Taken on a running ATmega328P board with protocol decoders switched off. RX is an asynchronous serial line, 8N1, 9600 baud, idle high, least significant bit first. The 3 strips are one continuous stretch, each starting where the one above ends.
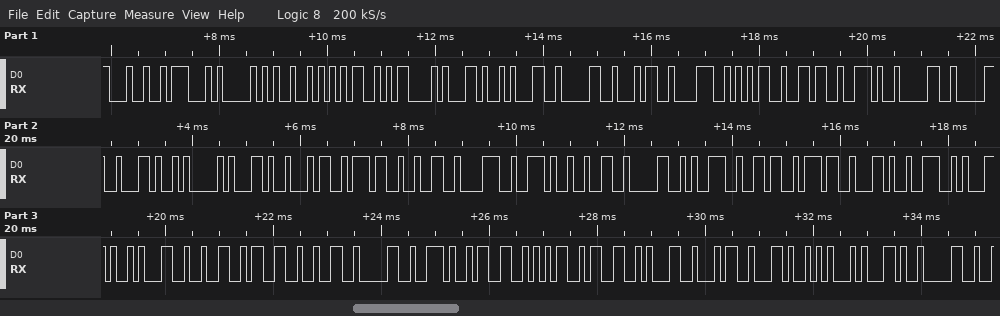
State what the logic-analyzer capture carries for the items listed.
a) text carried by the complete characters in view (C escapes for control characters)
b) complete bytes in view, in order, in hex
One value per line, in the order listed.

"$GPRMC,104856.00,A,4728.20967,N,12320.35314,E,0"
0x24 0x47 0x50 0x52 0x4D 0x43 0x2C 0x31 0x30 0x34 0x38 0x35 0x36 0x2E 0x30 0x30 0x2C 0x41 0x2C 0x34 0x37 0x32 0x38 0x2E 0x32 0x30 0x39 0x36 0x37 0x2C 0x4E 0x2C 0x31 0x32 0x33 0x32 0x30 0x2E 0x33 0x35 0x33 0x31 0x34 0x2C 0x45 0x2C 0x30
